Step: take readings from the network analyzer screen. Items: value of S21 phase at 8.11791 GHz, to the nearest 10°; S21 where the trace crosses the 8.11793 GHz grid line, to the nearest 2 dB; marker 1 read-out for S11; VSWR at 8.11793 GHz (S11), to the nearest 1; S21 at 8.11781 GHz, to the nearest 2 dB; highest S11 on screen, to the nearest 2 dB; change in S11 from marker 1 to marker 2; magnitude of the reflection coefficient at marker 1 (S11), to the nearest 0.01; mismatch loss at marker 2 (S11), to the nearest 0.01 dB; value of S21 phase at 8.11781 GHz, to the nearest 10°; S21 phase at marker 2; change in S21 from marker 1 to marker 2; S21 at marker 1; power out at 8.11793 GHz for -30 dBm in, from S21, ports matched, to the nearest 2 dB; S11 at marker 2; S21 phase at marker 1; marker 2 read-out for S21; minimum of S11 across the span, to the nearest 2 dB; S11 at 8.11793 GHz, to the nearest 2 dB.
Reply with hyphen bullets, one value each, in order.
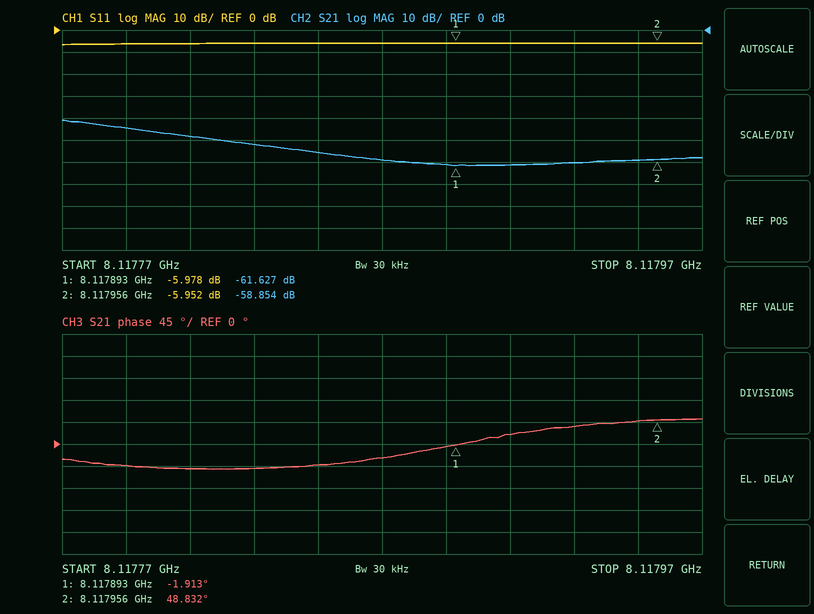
- 20°
- -60 dB
- -5.978 dB
- 3
- -48 dB
- -6 dB
- 0.026 dB
- 0.50
- 1.27 dB
- -50°
- 48.832°
- 2.773 dB
- -61.627 dB
- -90 dBm
- -5.952 dB
- -1.913°
- -58.854 dB
- -6 dB
- -6 dB
